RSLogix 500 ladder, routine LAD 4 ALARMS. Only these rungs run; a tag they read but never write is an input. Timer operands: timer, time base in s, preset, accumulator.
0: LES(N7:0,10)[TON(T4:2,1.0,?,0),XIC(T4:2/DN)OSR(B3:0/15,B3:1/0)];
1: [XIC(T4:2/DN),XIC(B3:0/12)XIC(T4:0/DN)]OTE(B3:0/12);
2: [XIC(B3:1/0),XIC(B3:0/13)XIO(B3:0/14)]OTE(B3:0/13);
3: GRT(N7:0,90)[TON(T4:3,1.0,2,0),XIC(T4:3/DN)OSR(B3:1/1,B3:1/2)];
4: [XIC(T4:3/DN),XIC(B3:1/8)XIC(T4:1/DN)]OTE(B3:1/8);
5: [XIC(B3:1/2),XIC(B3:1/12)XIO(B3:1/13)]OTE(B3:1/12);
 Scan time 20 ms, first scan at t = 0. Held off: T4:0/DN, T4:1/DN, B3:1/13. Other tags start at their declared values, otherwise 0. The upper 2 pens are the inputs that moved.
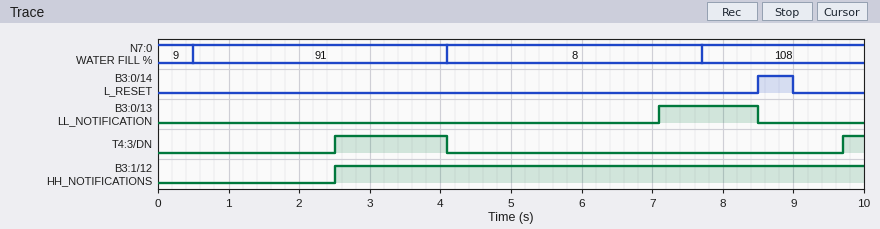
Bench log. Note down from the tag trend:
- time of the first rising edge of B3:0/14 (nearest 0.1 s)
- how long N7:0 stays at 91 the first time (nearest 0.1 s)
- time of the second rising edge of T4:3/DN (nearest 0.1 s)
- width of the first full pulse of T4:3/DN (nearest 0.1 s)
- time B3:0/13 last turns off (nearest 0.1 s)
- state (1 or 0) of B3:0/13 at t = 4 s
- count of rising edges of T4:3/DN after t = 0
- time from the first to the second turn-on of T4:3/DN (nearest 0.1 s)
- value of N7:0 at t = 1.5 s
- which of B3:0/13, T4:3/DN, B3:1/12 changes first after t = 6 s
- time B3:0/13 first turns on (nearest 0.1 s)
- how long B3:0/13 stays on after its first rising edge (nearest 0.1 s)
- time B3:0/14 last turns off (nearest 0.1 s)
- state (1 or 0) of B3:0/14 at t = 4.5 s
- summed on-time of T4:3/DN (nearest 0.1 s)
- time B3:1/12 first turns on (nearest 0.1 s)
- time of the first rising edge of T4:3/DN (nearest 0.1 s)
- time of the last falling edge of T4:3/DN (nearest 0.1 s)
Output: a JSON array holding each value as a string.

["8.5 s", "3.6 s", "9.7 s", "1.6 s", "8.5 s", "0", "2", "7.2 s", "91", "B3:0/13", "7.1 s", "1.4 s", "9.0 s", "0", "1.9 s", "2.5 s", "2.5 s", "4.1 s"]
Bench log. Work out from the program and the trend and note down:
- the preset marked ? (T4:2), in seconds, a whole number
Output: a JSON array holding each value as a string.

["3 s"]
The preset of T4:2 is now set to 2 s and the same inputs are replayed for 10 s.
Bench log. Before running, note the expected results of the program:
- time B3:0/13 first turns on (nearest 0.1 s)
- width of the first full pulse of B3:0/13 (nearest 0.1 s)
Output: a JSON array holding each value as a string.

["6.1 s", "2.4 s"]
